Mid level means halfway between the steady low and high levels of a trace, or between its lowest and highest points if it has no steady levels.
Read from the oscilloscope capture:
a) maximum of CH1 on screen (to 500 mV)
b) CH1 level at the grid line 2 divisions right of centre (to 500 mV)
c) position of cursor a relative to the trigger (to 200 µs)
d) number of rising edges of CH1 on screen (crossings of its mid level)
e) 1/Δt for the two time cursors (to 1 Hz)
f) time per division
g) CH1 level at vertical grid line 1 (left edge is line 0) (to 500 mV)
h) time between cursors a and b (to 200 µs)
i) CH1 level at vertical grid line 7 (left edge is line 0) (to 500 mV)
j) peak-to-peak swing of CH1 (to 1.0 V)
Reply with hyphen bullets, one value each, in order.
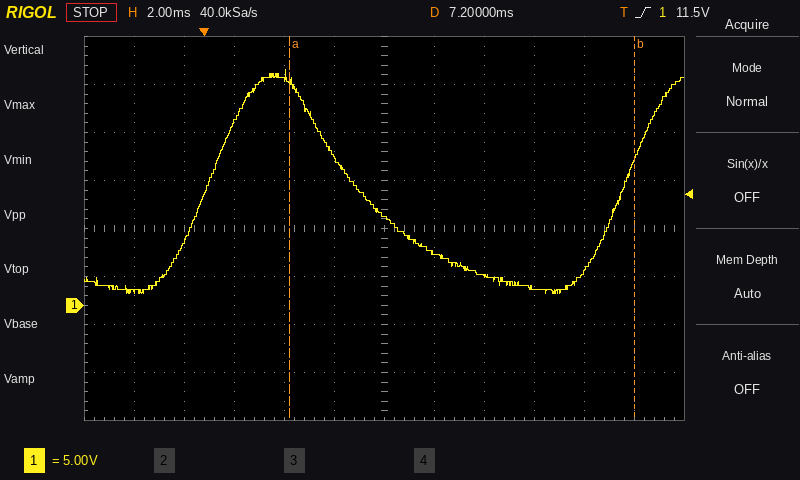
- 24.5 V
- 3.0 V
- +3.4 ms
- 2
- 72 Hz
- 2 ms
- 1.5 V
- 13.8 ms
- 5.5 V
- 23.0 V
